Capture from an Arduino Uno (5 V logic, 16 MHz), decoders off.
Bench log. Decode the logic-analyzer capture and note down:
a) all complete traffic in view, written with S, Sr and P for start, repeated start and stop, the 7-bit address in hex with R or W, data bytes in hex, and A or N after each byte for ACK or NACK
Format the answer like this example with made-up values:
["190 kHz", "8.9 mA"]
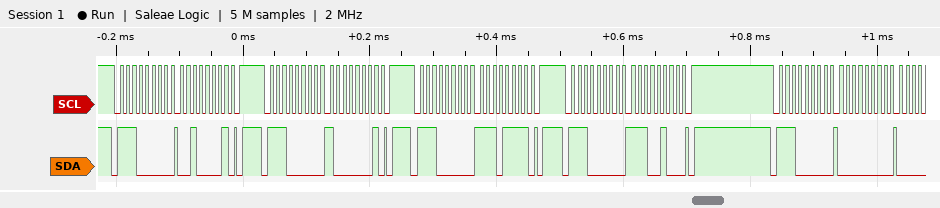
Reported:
["S 70W A 21 A P S 70W A 81 A P S 70W A EF A P S 70W A E4 A P S 70W A 00 A"]
